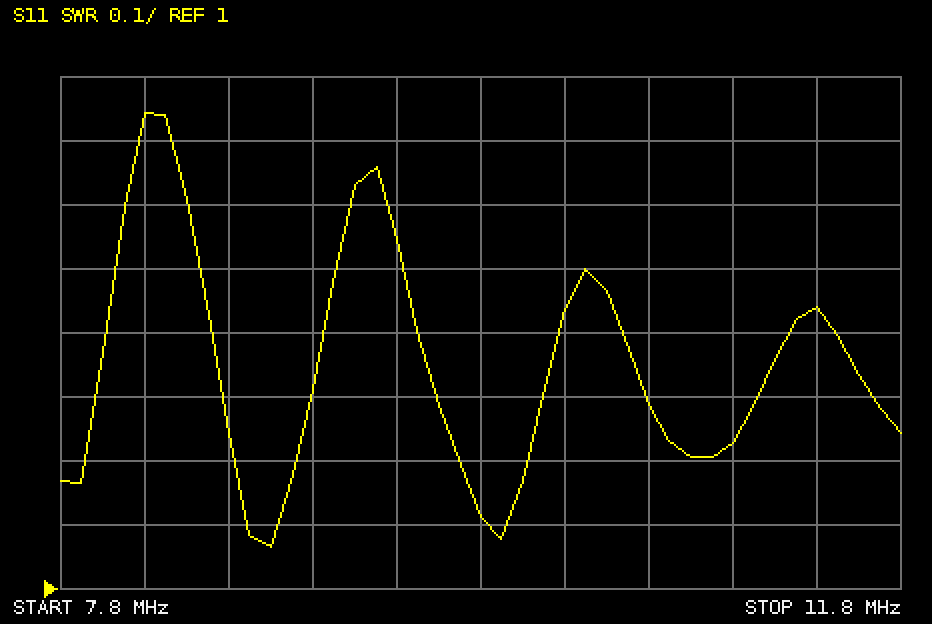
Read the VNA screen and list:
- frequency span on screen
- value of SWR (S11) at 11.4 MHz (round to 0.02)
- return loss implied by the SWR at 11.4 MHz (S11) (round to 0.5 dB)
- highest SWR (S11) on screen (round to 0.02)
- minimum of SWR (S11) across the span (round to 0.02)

4 MHz
1.44
15.0 dB
1.74
1.06
